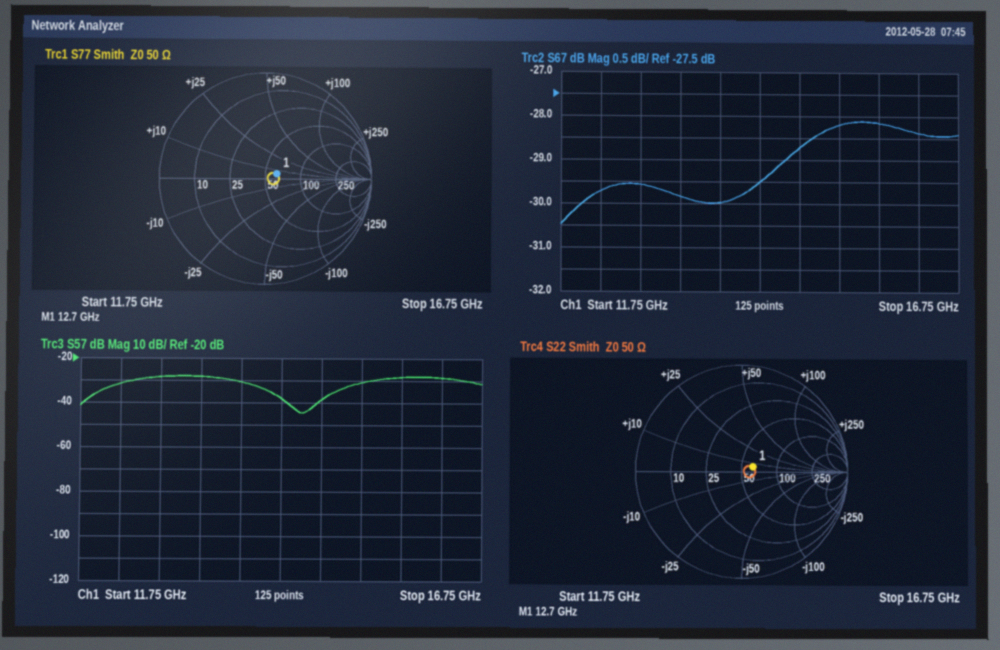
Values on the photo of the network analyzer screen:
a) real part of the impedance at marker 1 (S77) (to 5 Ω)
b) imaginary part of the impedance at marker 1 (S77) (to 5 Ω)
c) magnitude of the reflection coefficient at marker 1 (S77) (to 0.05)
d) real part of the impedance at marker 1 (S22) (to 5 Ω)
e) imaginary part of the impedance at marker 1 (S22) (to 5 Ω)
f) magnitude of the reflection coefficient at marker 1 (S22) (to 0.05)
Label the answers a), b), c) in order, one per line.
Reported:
a) 60 Ω
b) +5 Ω
c) 0.10
d) 60 Ω
e) +5 Ω
f) 0.10
